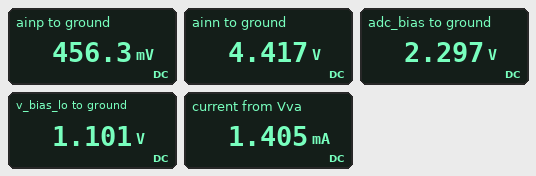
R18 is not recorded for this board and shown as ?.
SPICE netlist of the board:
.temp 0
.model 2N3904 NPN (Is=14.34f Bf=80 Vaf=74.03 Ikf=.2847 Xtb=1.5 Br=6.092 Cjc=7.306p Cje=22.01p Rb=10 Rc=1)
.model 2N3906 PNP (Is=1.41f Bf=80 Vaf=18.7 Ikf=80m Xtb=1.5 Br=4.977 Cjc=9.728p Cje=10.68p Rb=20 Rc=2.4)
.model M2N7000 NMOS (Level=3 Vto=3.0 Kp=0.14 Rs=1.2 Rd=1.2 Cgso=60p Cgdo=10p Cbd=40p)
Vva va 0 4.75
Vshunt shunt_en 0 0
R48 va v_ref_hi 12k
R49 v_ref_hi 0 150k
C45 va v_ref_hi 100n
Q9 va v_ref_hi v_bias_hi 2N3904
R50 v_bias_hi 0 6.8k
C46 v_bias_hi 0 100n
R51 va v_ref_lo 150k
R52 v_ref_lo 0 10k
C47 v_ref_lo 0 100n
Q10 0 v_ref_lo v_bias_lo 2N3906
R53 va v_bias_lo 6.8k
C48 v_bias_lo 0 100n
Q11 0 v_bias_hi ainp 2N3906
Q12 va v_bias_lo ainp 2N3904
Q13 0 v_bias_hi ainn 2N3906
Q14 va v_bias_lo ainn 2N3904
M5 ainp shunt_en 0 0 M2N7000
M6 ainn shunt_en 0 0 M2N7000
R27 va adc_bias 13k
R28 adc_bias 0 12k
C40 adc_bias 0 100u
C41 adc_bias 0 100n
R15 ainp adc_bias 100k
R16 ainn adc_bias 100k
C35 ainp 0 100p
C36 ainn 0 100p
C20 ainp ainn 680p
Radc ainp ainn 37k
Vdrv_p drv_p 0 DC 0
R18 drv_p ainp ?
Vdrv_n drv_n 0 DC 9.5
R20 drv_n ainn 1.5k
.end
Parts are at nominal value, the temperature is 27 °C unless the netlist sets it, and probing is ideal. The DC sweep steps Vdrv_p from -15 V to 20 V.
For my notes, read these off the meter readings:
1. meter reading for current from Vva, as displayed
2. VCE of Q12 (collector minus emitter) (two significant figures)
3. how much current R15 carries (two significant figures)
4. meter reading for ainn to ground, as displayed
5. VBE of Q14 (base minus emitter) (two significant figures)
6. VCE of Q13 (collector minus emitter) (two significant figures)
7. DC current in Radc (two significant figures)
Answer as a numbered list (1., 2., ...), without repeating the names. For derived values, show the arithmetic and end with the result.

1. 1.405 mA
2. 4.75 V - 456.3 mV = 4.3 V
3. (2.297 V - 456.3 mV) / 100 kΩ = 18 µA
4. 4.417 V
5. 1.101 V - 4.417 V = -3.3 V
6. 0 V - 4.417 V = -4.4 V
7. (4.417 V - 456.3 mV) / 37 kΩ = 110 µA
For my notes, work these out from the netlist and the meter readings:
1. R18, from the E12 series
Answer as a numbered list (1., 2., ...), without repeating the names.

1. 1.8 kΩ
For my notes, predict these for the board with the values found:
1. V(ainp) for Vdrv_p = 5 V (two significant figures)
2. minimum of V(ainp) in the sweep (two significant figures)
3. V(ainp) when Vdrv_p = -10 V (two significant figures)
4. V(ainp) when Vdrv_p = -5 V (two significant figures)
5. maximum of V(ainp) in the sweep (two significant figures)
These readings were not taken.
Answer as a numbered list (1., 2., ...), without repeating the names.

1. 4.4 V
2. 340 mV
3. 350 mV
4. 380 mV
5. 4.5 V
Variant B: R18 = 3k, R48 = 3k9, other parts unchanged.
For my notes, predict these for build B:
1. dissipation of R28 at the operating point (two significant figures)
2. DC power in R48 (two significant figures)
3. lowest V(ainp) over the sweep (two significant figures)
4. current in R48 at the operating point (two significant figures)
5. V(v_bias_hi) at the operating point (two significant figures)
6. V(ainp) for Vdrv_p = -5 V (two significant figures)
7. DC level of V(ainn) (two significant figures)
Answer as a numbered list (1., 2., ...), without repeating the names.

1. 450 µW
2. 5.7 µW
3. 360 mV
4. 38 µA
5. 3.9 V
6. 390 mV
7. 4.7 V
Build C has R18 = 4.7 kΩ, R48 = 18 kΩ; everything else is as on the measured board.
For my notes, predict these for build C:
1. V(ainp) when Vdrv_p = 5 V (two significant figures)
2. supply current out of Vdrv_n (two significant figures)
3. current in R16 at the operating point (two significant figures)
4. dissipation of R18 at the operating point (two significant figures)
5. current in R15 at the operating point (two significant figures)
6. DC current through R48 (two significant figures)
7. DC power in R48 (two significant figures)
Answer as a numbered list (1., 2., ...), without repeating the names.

1. 4.2 V
2. 3.5 mA
3. 19 µA
4. 66 µW
5. 17 µA
6. 34 µA
7. 21 µW
